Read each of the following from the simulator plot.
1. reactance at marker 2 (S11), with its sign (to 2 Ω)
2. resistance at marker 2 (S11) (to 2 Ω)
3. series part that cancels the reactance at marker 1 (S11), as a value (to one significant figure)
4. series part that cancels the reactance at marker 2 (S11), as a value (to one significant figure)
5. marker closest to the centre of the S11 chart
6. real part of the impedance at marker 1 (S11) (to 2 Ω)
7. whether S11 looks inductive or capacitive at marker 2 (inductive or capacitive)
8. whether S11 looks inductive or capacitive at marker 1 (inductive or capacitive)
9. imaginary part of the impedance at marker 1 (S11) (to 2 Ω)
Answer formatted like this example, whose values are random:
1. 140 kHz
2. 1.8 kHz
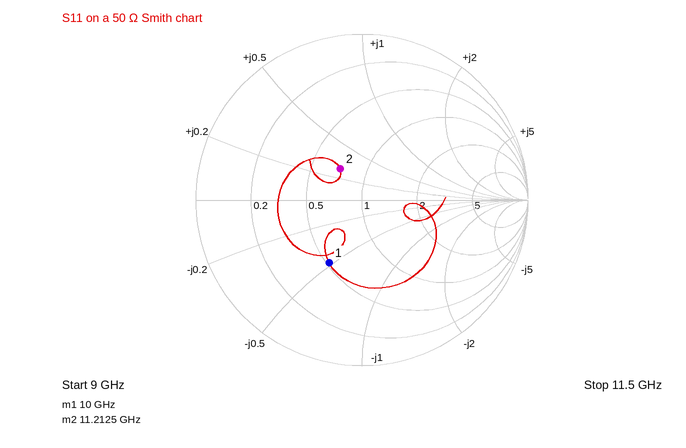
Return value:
1. +14 Ω
2. 36 Ω
3. 400 pH
4. 1.0 pF
5. marker 2
6. 26 Ω
7. inductive
8. capacitive
9. -24 Ω
